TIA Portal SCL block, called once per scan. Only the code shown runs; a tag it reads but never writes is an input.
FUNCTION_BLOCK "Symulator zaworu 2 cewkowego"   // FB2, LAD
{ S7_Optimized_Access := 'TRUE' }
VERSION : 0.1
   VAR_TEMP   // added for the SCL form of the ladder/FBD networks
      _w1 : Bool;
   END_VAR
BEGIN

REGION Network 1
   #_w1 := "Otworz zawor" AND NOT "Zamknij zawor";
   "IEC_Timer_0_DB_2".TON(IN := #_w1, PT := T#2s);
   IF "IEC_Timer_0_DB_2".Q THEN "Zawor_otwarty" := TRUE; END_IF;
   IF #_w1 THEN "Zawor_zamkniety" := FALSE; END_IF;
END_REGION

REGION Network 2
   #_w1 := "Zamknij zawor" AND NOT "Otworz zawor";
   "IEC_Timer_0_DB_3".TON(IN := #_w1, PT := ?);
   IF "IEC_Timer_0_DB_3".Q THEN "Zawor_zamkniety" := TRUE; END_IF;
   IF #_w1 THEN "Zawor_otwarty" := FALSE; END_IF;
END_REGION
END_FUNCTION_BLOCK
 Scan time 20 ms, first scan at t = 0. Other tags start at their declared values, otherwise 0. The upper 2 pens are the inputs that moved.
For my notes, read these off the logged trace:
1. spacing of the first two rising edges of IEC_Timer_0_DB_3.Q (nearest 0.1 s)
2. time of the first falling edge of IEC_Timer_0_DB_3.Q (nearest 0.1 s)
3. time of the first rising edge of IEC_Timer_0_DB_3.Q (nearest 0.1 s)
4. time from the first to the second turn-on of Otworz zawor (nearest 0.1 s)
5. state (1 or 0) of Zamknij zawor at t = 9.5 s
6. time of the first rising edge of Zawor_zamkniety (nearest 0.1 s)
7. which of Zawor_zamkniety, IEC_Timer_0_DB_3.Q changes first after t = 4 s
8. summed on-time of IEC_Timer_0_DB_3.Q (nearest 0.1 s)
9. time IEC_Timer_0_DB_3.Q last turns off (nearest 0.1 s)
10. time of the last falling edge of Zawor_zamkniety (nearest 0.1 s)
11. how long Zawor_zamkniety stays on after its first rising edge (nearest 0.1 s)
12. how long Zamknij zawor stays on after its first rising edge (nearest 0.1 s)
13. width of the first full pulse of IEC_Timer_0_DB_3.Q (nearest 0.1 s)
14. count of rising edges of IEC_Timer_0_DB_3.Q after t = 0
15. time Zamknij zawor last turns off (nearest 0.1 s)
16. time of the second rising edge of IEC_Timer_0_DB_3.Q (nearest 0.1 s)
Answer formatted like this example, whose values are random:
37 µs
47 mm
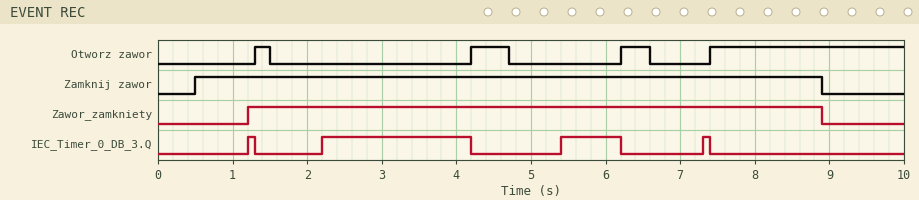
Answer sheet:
1.0 s
1.3 s
1.2 s
2.9 s
0
1.2 s
IEC_Timer_0_DB_3.Q
3.0 s
7.4 s
8.9 s
7.7 s
8.4 s
0.1 s
4
8.9 s
2.2 s
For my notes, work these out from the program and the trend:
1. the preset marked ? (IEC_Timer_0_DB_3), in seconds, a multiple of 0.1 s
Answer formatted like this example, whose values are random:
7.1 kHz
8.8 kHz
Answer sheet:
0.7 s
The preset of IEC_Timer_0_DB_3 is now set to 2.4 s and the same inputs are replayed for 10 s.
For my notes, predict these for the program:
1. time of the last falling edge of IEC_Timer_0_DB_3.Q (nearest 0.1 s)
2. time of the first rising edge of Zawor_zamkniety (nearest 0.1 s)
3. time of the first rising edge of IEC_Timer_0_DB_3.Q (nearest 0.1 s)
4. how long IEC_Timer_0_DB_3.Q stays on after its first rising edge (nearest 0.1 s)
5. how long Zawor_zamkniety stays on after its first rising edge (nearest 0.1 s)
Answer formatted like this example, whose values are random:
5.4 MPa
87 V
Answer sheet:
4.2 s
3.9 s
3.9 s
0.3 s
5.0 s
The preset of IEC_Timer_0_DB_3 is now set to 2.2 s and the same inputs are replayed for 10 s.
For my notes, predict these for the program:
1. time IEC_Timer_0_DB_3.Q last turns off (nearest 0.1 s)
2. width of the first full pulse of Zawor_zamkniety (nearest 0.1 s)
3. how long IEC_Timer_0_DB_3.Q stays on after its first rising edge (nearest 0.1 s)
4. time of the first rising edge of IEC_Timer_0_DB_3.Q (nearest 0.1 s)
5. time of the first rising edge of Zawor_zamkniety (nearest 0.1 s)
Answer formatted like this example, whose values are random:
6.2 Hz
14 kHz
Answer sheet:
4.2 s
5.2 s
0.5 s
3.7 s
3.7 s
